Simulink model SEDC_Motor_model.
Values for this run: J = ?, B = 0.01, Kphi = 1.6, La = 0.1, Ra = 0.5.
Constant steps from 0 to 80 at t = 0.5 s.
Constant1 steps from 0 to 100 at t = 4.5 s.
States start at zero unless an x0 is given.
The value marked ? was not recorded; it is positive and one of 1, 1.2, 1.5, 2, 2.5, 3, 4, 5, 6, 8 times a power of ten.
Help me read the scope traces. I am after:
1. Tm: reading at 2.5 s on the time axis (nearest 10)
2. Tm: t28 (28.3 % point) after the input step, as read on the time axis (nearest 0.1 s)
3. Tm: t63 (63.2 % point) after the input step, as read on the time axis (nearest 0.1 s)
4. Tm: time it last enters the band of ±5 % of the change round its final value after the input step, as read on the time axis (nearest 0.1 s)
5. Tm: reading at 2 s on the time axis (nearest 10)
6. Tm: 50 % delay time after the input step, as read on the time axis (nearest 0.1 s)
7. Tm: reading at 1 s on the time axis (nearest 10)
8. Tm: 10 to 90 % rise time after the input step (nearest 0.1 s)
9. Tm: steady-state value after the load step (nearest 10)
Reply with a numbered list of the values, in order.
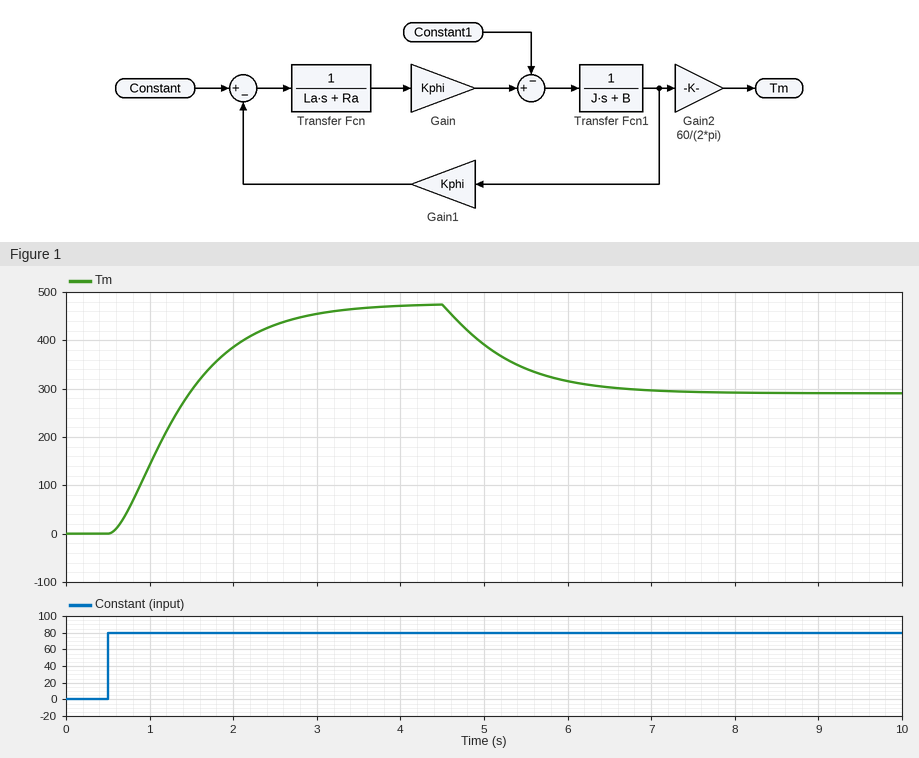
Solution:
1. 430
2. 1.0 s
3. 1.5 s
4. 2.9 s
5. 390
6. 1.3 s
7. 140
8. 1.7 s
9. 290
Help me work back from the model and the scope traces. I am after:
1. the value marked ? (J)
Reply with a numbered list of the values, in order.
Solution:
1. 5
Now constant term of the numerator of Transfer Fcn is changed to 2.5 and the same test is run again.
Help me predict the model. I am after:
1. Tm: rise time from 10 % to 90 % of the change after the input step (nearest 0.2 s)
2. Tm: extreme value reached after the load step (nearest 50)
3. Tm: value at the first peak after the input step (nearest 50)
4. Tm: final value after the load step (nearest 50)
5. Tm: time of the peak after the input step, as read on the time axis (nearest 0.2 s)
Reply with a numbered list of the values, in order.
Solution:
1. 0.6 s
2. 400
3. 500
4. 400
5. 1.8 s
